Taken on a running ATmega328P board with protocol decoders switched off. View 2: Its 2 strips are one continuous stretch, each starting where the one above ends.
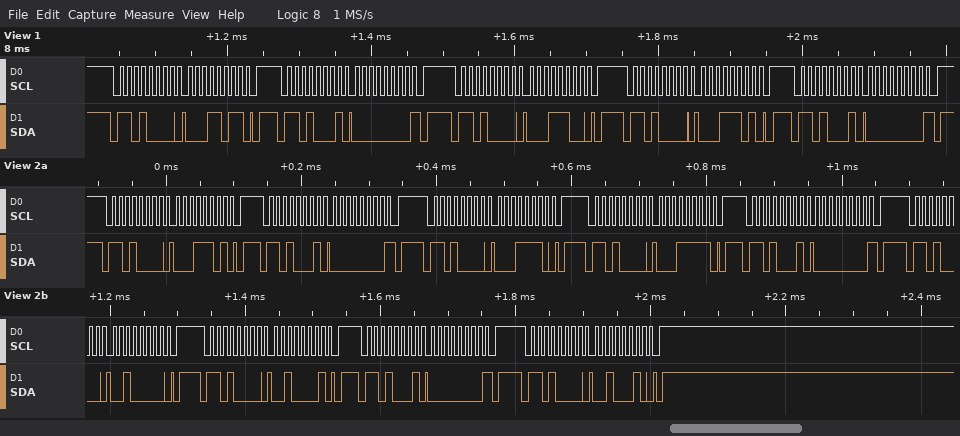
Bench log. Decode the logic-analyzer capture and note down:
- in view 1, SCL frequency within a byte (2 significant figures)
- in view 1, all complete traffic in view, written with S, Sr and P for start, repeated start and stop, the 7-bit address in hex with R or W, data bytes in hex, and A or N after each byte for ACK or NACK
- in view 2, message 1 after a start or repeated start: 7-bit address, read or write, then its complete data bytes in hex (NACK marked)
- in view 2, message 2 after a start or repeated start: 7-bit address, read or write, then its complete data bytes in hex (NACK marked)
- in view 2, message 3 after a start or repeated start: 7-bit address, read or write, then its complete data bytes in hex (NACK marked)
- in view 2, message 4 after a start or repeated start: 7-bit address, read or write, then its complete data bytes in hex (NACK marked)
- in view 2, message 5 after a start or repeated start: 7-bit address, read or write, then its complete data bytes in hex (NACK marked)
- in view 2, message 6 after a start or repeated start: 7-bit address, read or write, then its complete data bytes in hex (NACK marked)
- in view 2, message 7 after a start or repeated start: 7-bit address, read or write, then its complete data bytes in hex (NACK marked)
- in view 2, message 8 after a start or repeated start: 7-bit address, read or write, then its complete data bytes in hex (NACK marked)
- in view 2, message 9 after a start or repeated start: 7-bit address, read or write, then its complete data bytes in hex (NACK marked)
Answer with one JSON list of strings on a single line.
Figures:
["100 kHz", "S 68W A 1B A P S 68R A 00 N P S 68W A 1C A P S 68W A 1D A P S 68R A 00 N P", "0x68 write: 1D", "0x68 read: 00 NACK", "0x68 write: 1E", "0x68 write: 1F", "0x68 read: 00 NACK", "0x68 write: 20", "0x68 write: 21", "0x68 read: 00 NACK", "0x68 write: 22"]
